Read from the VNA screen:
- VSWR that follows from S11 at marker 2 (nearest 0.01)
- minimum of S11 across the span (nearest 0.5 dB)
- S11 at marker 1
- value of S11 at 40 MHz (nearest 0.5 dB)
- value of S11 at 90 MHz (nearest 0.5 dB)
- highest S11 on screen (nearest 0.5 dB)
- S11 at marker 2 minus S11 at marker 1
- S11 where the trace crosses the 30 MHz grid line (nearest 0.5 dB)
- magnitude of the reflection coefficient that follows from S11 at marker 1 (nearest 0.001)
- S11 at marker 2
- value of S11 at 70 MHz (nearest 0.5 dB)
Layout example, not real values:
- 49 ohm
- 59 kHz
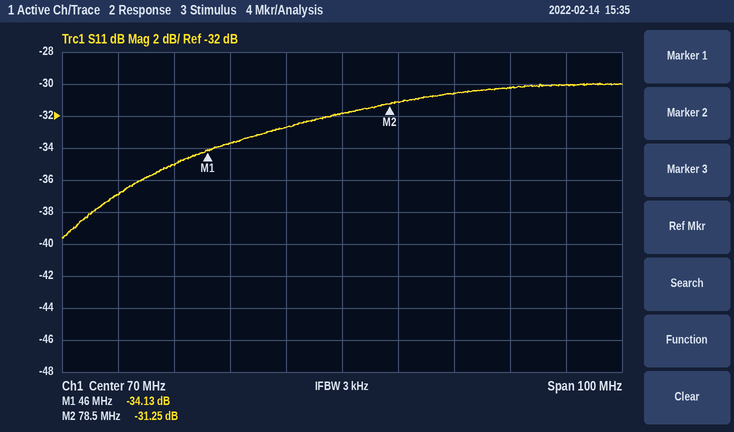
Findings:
- 1.06
- -39.5 dB
- -34.13 dB
- -35.0 dB
- -30.5 dB
- -30.0 dB
- 2.88 dB
- -37.0 dB
- 0.020
- -31.25 dB
- -32.0 dB
